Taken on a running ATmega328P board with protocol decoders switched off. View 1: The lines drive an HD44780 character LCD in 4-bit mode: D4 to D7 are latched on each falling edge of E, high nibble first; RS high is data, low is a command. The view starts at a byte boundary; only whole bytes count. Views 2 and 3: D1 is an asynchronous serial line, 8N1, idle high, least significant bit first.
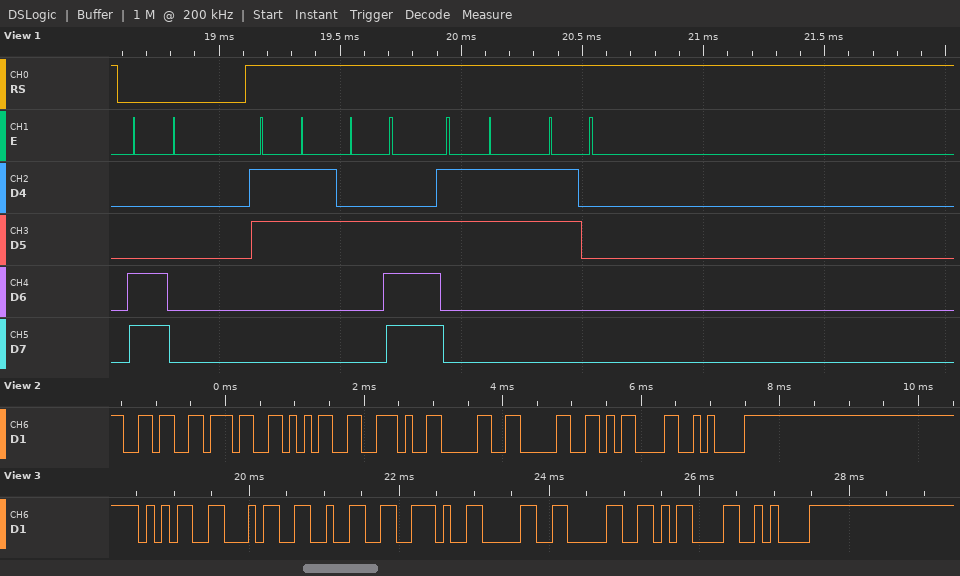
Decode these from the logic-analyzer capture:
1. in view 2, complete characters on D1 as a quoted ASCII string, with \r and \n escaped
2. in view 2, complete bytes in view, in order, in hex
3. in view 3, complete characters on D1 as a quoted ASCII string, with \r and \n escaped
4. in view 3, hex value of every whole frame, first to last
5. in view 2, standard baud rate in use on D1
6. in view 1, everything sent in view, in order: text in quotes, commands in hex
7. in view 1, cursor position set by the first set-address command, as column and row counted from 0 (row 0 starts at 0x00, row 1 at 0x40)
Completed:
"675.00\r\n"
36 37 35 2E 30 30 0D 0A
"542.00\r\n"
35 34 32 2E 30 30 0D 0A
9600 baud
0xC0 "3.30"
column 0, row 1
